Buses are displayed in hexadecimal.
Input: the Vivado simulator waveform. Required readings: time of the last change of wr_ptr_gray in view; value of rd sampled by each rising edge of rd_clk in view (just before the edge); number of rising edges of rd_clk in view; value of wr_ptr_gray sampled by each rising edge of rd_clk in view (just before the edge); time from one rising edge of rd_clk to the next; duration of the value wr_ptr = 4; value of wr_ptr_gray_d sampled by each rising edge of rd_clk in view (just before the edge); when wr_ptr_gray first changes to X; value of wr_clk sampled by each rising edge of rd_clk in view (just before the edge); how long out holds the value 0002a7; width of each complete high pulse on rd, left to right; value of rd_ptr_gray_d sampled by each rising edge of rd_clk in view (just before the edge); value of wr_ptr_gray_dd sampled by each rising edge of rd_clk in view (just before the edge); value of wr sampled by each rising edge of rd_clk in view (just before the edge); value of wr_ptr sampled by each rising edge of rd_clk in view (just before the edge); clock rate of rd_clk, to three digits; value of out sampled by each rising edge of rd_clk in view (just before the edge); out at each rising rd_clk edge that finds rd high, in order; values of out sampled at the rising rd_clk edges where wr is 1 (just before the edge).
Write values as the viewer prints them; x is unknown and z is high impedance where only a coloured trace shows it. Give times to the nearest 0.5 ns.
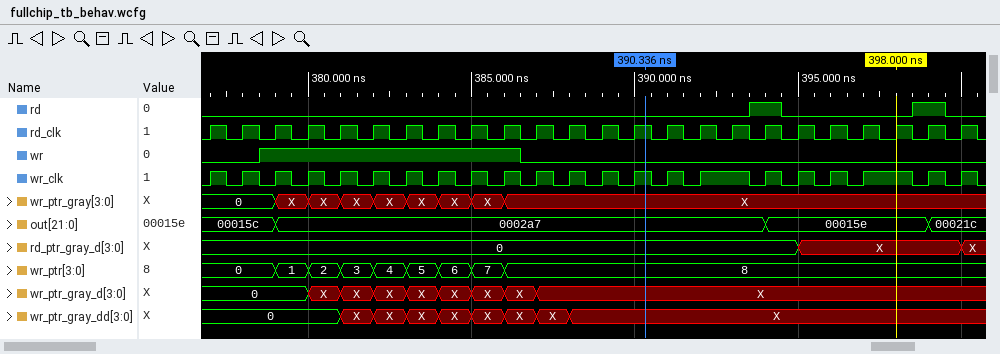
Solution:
386 ns
0 0 0 0 0 0 0 0 0 0 0 0 0 0 0 0 0 1 0 0 0 0 1 0
24
0, 0, 0, X, X, X, X, X, X, X, X, X, X, X, X, X, X, X, X, X, X, X, X, X
1 ns
1 ns
0, 0, 0, 0, X, X, X, X, X, X, X, X, X, X, X, X, X, X, X, X, X, X, X, X
379 ns
0 0 0 0 0 0 0 0 0 0 0 0 0 0 0 0 1 0 0 0 0 1 0 0
15 ns
1 ns, 1 ns
0, 0, 0, 0, 0, 0, 0, 0, 0, 0, 0, 0, 0, 0, 0, 0, 0, 0, 0, X, X, X, X, X
0, 0, 0, 0, 0, X, X, X, X, X, X, X, X, X, X, X, X, X, X, X, X, X, X, X
0 0 1 1 1 1 1 1 1 1 0 0 0 0 0 0 0 0 0 0 0 0 0 0
0, 0, 0, 1, 2, 3, 4, 5, 6, 7, 8, 8, 8, 8, 8, 8, 8, 8, 8, 8, 8, 8, 8, 8
1.00 GHz
00015c, 00015c, 00015c, 0002a7, 0002a7, 0002a7, 0002a7, 0002a7, 0002a7, 0002a7, 0002a7, 0002a7, 0002a7, 0002a7, 0002a7, 0002a7, 0002a7, 0002a7, 00015e, 00015e, 00015e, 00015e, 00015e, 00021c
0002a7, 00015e
00015c, 0002a7, 0002a7, 0002a7, 0002a7, 0002a7, 0002a7, 0002a7
